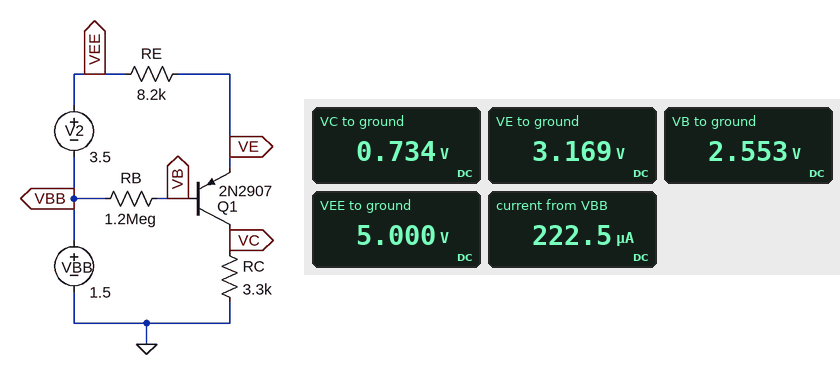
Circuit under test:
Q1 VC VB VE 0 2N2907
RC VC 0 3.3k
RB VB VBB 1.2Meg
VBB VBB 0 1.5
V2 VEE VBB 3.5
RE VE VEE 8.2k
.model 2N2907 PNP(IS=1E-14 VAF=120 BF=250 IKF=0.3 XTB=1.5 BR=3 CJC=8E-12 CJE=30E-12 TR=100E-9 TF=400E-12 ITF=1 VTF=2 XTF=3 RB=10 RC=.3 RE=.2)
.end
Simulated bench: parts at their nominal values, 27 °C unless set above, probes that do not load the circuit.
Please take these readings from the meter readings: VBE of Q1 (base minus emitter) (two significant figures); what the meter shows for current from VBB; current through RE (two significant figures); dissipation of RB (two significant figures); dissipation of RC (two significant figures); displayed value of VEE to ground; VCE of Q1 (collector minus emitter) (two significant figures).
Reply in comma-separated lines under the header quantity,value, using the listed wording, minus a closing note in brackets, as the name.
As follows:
quantity,value
VBE of Q1 (base minus emitter),-620 mV
what the meter shows for current from VBB,222.5 µA
current through RE,220 µA
dissipation of RB,920 nW
dissipation of RC,160 µW
displayed value of VEE to ground,5.000 V
VCE of Q1 (collector minus emitter),-2.4 V
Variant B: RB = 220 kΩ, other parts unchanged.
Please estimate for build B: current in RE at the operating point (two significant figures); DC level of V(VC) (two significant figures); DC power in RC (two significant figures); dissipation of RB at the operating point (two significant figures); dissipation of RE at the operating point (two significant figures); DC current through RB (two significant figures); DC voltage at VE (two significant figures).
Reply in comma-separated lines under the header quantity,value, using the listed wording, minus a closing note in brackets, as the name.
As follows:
quantity,value
current in RE at the operating point,320 µA
DC level of V(VC),1.0 V
DC power in RC,330 µW
dissipation of RB at the operating point,350 nW
dissipation of RE at the operating point,820 µW
DC current through RB,1.3 µA
DC voltage at VE,2.4 V
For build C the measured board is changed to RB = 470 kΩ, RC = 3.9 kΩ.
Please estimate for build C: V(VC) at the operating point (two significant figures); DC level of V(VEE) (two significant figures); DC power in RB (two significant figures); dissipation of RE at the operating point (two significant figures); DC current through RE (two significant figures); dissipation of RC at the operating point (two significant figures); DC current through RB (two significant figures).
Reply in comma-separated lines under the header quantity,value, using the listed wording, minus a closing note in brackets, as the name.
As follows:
quantity,value
V(VC) at the operating point,1.1 V
DC level of V(VEE),5.0 V
DC power in RB,600 nW
dissipation of RE at the operating point,670 µW
DC current through RE,290 µA
dissipation of RC at the operating point,320 µW
DC current through RB,1.1 µA
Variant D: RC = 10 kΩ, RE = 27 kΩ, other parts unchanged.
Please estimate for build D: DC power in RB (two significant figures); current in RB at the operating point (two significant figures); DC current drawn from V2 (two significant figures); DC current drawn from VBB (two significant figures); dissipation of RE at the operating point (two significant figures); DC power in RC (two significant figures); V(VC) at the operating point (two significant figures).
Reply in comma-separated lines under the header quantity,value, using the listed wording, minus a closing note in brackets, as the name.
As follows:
quantity,value
DC power in RB,160 nW
current in RB at the operating point,360 nA
DC current drawn from V2,92 µA
DC current drawn from VBB,91 µA
dissipation of RE at the operating point,230 µW
DC power in RC,83 µW
V(VC) at the operating point,910 mV
